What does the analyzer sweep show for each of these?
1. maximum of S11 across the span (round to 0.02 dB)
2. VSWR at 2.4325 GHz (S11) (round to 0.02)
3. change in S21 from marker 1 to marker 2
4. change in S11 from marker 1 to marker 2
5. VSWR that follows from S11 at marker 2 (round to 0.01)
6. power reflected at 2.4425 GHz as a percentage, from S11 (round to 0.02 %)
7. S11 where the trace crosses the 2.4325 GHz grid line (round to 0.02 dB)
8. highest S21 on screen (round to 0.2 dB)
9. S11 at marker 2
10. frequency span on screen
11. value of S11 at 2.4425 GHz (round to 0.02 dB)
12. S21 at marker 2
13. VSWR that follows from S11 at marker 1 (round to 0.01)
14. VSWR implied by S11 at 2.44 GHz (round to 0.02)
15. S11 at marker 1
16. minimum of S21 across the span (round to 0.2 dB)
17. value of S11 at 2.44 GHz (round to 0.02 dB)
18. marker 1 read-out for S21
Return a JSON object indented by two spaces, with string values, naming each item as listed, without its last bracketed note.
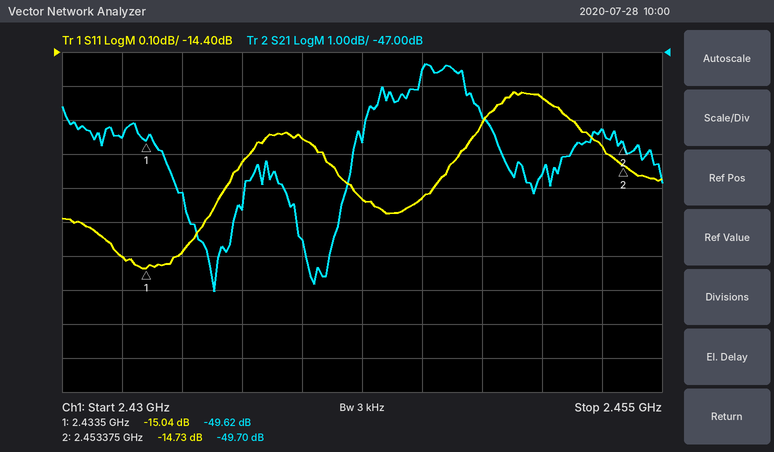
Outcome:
{
  "maximum of S11 across the span": "-14.52 dB",
  "VSWR at 2.4325 GHz (S11)": "1.44",
  "change in S21 from marker 1 to marker 2": "-0.08 dB",
  "change in S11 from marker 1 to marker 2": "0.31 dB",
  "VSWR that follows from S11 at marker 2": "1.45",
  "power reflected at 2.4425 GHz as a percentage, from S11": "3.28 %",
  "S11 where the trace crosses the 2.4325 GHz grid line": "-15.00 dB",
  "highest S21 on screen": "-47.4 dB",
  "S11 at marker 2": "-14.73 dB",
  "frequency span on screen": "25 MHz",
  "value of S11 at 2.4425 GHz": "-14.84 dB",
  "S21 at marker 2": "-49.70 dB",
  "VSWR that follows from S11 at marker 1": "1.43",
  "VSWR implied by S11 at 2.44 GHz": "1.46",
  "S11 at marker 1": "-15.04 dB",
  "minimum of S21 across the span": "-54.0 dB",
  "value of S11 at 2.44 GHz": "-14.66 dB",
  "marker 1 read-out for S21": "-49.62 dB"
}
